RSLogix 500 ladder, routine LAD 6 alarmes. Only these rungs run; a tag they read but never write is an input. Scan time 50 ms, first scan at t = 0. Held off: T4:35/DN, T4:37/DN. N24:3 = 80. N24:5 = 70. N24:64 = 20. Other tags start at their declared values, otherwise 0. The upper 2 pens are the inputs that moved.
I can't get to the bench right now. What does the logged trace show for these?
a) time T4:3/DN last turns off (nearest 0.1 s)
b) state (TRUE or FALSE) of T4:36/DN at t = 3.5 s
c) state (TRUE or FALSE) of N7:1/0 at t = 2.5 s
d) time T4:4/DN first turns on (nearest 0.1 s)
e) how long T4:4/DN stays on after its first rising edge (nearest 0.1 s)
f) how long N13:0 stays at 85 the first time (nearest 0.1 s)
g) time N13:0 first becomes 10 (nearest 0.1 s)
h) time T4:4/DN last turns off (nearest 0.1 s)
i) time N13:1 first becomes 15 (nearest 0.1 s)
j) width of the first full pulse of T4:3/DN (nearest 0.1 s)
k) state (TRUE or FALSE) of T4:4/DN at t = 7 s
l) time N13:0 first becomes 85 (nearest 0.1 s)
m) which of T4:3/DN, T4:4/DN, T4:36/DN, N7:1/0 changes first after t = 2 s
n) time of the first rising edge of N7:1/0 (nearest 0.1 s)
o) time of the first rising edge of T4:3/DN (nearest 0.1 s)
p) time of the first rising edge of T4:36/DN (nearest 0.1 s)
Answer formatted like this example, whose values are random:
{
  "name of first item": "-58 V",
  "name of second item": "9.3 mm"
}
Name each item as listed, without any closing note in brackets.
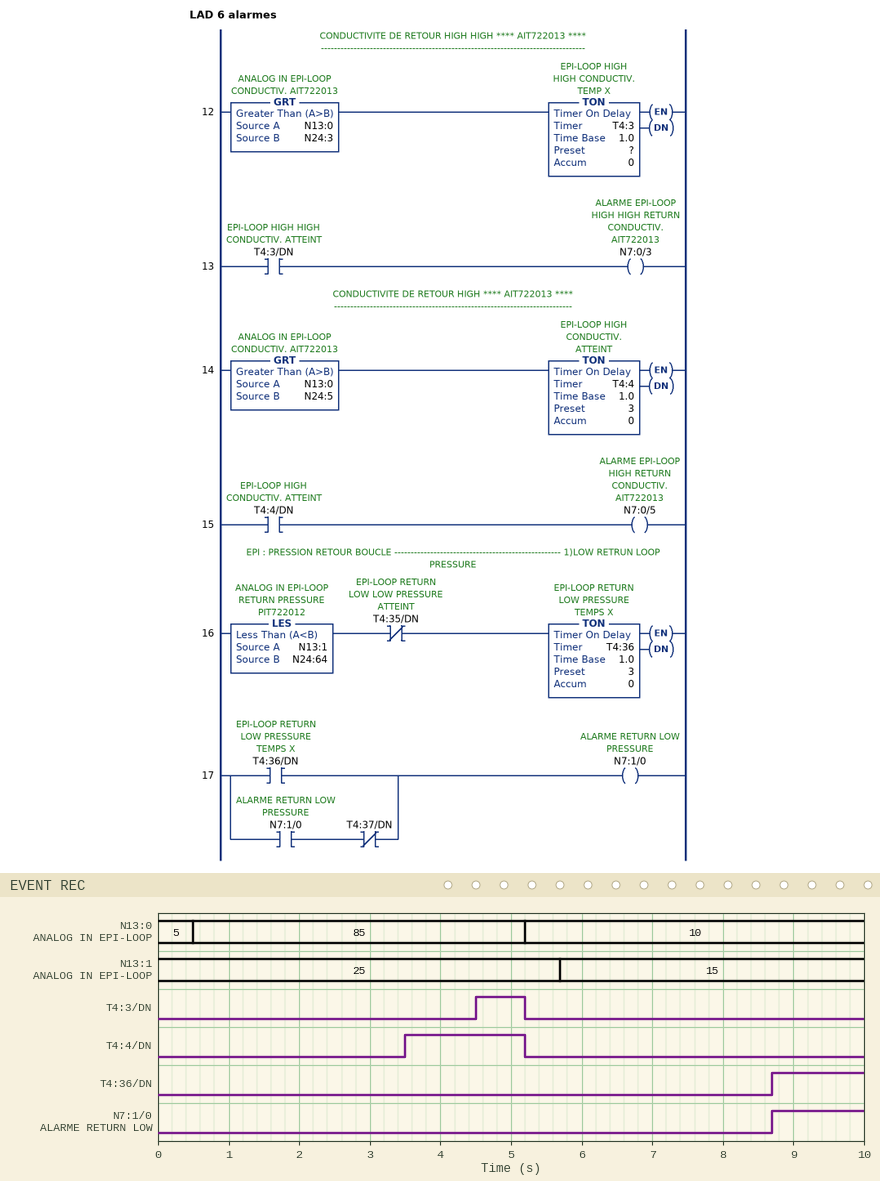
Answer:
{
  "time T4:3/DN last turns off": "5.2 s",
  "state (TRUE or FALSE) of T4:36/DN at t = 3.5 s": "FALSE",
  "state (TRUE or FALSE) of N7:1/0 at t = 2.5 s": "FALSE",
  "time T4:4/DN first turns on": "3.5 s",
  "how long T4:4/DN stays on after its first rising edge": "1.7 s",
  "how long N13:0 stays at 85 the first time": "4.7 s",
  "time N13:0 first becomes 10": "5.2 s",
  "time T4:4/DN last turns off": "5.2 s",
  "time N13:1 first becomes 15": "5.7 s",
  "width of the first full pulse of T4:3/DN": "0.7 s",
  "state (TRUE or FALSE) of T4:4/DN at t = 7 s": "FALSE",
  "time N13:0 first becomes 85": "0.5 s",
  "which of T4:3/DN, T4:4/DN, T4:36/DN, N7:1/0 changes first after t = 2 s": "T4:4/DN",
  "time of the first rising edge of N7:1/0": "8.7 s",
  "time of the first rising edge of T4:3/DN": "4.5 s",
  "time of the first rising edge of T4:36/DN": "8.7 s"
}
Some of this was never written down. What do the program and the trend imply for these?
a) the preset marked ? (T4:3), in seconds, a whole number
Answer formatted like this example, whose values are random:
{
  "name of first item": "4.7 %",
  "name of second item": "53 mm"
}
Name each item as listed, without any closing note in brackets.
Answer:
{
  "the preset marked ? (T4:3), in seconds, a whole number": "4 s"
}
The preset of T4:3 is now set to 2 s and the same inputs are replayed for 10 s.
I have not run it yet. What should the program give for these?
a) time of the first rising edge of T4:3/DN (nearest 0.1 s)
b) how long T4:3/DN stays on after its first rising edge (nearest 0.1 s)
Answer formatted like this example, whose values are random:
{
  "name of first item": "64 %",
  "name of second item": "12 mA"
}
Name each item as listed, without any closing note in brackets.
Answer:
{
  "time of the first rising edge of T4:3/DN": "2.5 s",
  "how long T4:3/DN stays on after its first rising edge": "2.7 s"
}
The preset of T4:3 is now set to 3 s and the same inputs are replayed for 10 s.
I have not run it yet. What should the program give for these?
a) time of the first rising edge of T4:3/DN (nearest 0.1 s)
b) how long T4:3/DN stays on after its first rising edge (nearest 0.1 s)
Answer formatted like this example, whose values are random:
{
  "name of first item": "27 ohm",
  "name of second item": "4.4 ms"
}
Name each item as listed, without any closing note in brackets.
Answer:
{
  "time of the first rising edge of T4:3/DN": "3.5 s",
  "how long T4:3/DN stays on after its first rising edge": "1.7 s"
}
